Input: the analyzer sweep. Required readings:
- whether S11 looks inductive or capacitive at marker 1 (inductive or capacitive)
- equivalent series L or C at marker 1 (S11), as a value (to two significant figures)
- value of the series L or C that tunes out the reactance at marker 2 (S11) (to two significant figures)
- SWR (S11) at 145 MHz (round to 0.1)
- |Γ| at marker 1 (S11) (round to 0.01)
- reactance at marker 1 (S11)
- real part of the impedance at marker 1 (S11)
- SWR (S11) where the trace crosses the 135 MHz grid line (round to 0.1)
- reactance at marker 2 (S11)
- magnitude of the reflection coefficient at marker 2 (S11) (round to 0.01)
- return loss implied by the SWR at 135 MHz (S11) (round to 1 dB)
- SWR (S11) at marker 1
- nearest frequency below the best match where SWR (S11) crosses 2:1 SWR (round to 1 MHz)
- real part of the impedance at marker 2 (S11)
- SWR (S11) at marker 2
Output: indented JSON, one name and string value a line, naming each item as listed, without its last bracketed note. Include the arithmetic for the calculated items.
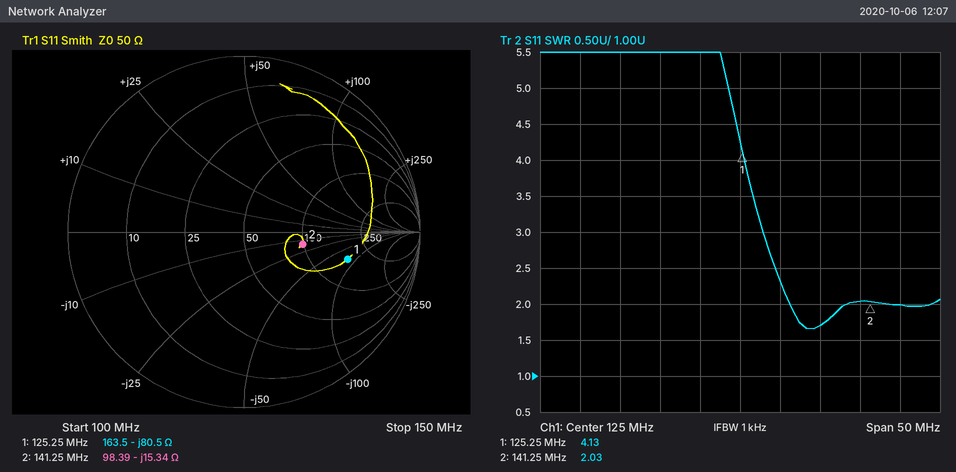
{
  "whether S11 looks inductive or capacitive at marker 1": "capacitive",
  "equivalent series L or C at marker 1 (S11), as a value": "C = 1/(2π × 125.25 MHz × 80.5 Ω) ≈ 16 pF",
  "value of the series L or C that tunes out the reactance at marker 2 (S11)": "L = 15.34 Ω/(2π × 141.25 MHz) ≈ 17 nH",
  "SWR (S11) at 145 MHz": "2.0",
  "|Γ| at marker 1 (S11)": "0.61",
  "reactance at marker 1": "-80.5 Ω",
  "real part of the impedance at marker 1": "163.5 Ω",
  "SWR (S11) where the trace crosses the 135 MHz grid line": "1.7",
  "reactance at marker 2": "-15.34 Ω",
  "magnitude of the reflection coefficient at marker 2 (S11)": "0.34",
  "return loss implied by the SWR at 135 MHz (S11)": "−20 log10((1.7 − 1)/(1.7 + 1)) ≈ 12 dB",
  "SWR (S11) at marker 1": "4.13",
  "nearest frequency below the best match where SWR (S11) crosses 2:1 SWR": "131 MHz",
  "real part of the impedance at marker 2": "98.39 Ω",
  "SWR (S11) at marker 2": "2.03"
}
